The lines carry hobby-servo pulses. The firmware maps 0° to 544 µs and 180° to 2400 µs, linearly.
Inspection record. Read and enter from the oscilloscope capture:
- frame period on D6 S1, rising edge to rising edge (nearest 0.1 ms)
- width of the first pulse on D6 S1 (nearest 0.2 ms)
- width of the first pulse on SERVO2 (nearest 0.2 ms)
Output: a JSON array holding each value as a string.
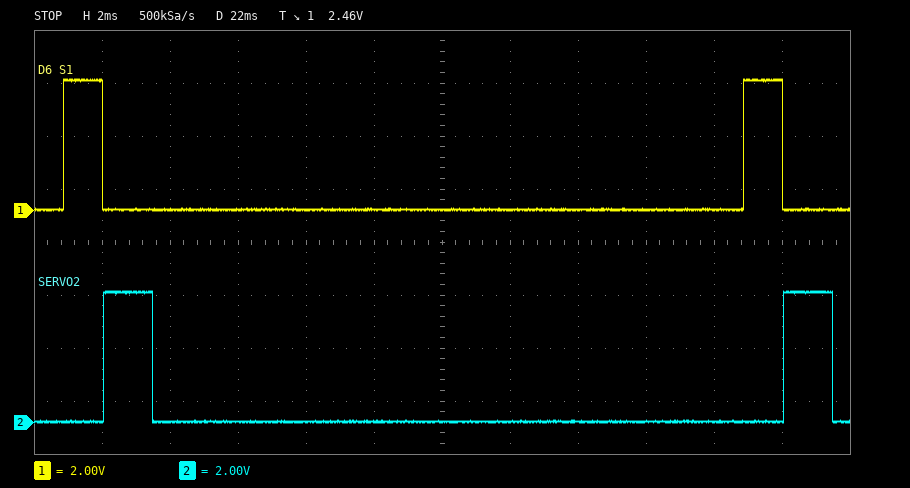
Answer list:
["20.0 ms", "1.2 ms", "1.4 ms"]
